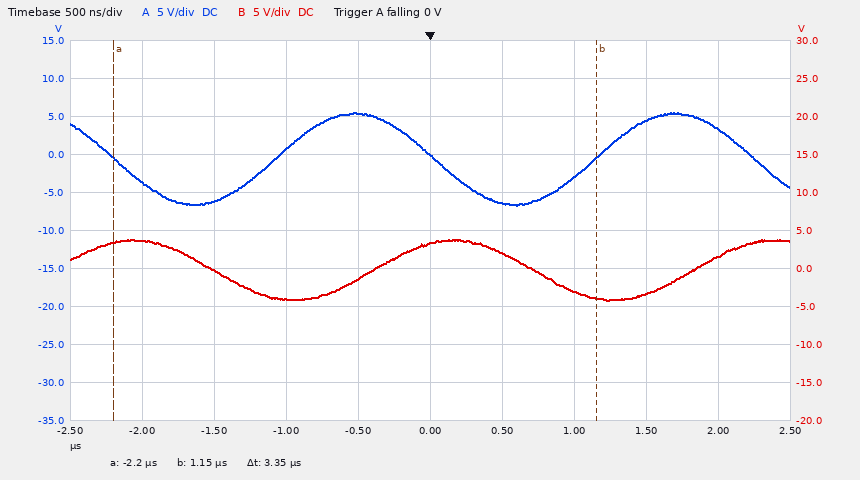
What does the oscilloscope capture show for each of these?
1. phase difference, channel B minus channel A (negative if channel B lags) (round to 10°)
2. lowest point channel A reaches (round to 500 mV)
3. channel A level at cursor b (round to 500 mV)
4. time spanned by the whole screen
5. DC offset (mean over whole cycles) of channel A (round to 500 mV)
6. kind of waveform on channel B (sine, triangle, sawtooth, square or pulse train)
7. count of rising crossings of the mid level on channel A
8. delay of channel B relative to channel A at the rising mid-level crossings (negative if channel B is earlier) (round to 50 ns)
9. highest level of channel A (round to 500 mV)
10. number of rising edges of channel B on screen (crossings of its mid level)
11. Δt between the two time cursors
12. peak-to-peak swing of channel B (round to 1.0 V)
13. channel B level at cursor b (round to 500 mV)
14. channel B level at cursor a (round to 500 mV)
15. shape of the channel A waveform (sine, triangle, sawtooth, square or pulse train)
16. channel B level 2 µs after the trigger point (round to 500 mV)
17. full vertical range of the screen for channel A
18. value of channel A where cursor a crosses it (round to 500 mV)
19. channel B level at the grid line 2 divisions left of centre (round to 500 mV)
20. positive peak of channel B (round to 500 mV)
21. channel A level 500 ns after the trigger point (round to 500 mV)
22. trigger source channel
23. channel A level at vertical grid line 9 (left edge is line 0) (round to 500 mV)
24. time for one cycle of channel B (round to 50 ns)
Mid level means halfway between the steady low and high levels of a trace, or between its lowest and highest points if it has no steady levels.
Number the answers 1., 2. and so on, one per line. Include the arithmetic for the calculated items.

1. −360° × (+700 ns) / 2.20 µs ≈ -115°, so -110° to the nearest 10°
2. -6.5 V
3. -500 mV
4. 5 µs
5. (5.5 V + (-6.5 V)) / 2 ≈ -500 mV
6. sine
7. 2
8. +700 ns
9. 5.5 V
10. 2
11. 3.35 µs
12. 8.0 V
13. -4.0 V
14. 3.5 V
15. sine
16. 1.5 V
17. 50 V
18. -500 mV
19. -4.0 V
20. 4.0 V
21. -6.5 V
22. channel A
23. 3.5 V
24. 2.20 µs
